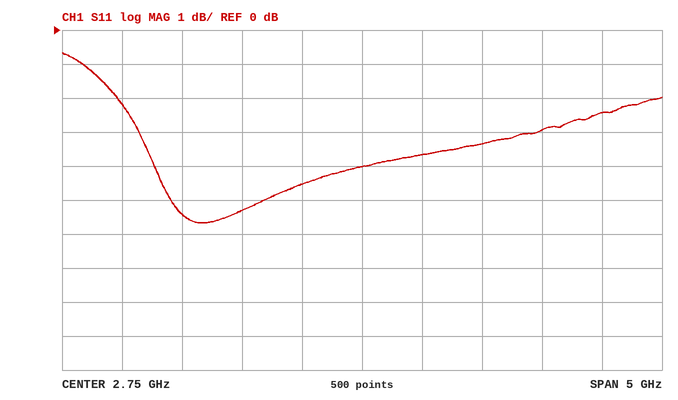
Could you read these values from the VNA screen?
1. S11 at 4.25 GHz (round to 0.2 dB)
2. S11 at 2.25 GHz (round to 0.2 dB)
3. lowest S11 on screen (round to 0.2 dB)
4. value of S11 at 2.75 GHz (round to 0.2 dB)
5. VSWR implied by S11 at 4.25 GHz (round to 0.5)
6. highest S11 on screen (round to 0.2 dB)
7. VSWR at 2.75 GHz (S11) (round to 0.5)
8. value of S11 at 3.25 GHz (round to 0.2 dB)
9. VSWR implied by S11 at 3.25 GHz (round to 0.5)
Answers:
-3.0 dB
-4.6 dB
-5.6 dB
-4.0 dB
6.0
-0.6 dB
4.5
-3.6 dB
5.0
